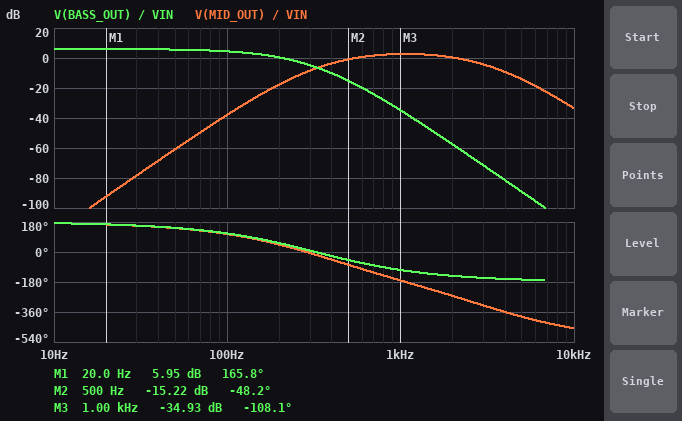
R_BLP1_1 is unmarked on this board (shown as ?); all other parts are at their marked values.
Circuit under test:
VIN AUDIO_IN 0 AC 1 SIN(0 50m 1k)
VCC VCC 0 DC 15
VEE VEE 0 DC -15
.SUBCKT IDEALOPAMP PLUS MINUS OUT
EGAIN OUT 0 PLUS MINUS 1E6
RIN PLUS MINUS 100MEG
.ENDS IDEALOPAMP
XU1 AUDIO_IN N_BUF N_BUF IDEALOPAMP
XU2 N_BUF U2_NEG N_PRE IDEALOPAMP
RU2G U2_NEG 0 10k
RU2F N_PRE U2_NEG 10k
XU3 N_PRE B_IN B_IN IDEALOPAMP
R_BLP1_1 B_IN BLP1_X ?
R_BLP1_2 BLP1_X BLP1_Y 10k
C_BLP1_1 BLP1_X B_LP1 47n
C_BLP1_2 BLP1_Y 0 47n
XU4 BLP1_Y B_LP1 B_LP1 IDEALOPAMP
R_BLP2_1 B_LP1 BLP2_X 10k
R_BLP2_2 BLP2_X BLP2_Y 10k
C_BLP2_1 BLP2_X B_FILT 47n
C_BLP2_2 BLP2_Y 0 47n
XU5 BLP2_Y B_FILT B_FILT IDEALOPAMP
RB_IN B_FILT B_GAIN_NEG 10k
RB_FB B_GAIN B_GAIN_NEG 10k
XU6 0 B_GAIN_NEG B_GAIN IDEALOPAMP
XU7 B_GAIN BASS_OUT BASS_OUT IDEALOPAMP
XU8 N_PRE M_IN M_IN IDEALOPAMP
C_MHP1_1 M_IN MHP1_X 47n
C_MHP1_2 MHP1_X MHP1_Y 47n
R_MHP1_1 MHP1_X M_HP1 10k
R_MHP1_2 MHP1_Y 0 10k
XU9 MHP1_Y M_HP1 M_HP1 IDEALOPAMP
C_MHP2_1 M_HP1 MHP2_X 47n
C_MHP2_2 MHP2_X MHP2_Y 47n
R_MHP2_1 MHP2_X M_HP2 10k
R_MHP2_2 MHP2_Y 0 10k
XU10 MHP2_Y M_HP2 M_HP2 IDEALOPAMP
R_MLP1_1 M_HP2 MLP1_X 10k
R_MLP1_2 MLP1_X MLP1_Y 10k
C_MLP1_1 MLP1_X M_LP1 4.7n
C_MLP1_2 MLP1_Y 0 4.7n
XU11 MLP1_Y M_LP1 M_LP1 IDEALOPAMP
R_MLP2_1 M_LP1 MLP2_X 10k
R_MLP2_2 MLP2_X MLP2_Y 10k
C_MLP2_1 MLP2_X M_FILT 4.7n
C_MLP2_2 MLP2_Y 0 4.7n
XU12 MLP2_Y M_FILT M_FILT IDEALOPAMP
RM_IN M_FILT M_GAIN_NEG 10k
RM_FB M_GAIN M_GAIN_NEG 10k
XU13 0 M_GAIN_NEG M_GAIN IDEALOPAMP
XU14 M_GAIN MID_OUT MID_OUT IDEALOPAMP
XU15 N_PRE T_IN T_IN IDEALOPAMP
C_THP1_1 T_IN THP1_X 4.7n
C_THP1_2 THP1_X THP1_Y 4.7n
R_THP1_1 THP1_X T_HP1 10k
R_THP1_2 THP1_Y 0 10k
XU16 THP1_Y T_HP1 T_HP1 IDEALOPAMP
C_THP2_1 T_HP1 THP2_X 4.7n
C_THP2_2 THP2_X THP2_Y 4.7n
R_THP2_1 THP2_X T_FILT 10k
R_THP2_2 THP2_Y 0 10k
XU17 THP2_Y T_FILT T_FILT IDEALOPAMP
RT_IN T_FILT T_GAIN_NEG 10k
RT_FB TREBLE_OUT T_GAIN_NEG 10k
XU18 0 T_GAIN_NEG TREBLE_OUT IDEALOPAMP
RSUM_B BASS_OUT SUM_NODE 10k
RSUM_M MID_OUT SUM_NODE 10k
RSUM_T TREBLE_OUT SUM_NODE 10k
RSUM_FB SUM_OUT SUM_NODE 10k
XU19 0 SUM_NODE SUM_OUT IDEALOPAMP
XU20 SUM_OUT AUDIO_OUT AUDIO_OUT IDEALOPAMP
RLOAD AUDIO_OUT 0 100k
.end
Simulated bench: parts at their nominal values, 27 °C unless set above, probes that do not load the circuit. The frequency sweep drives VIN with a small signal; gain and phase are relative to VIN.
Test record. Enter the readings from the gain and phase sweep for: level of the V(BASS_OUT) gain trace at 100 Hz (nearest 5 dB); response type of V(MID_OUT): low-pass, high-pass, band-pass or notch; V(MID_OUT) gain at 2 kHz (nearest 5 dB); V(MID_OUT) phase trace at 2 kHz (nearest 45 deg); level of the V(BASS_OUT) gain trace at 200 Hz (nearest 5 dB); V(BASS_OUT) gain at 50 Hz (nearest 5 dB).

5 dB
band-pass
0 dB
-270 deg
0 dB
5 dB
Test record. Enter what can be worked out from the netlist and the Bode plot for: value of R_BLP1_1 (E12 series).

12 kΩ
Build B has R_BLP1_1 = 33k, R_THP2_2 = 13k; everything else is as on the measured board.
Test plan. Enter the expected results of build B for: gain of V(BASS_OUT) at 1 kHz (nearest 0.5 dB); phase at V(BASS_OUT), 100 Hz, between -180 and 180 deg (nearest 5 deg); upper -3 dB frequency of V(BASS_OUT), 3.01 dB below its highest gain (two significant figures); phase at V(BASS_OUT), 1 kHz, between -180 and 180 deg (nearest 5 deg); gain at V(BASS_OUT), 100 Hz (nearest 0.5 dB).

-43.5 dB
85 deg
84 Hz
-120 deg
2.0 dB
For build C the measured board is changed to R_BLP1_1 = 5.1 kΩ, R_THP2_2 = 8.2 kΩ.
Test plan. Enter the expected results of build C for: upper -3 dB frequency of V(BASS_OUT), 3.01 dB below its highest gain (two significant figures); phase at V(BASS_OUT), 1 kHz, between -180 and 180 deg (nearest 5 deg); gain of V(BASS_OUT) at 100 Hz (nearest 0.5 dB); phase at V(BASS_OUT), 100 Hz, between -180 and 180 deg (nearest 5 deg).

160 Hz
-90 deg
5.0 dB
120 deg
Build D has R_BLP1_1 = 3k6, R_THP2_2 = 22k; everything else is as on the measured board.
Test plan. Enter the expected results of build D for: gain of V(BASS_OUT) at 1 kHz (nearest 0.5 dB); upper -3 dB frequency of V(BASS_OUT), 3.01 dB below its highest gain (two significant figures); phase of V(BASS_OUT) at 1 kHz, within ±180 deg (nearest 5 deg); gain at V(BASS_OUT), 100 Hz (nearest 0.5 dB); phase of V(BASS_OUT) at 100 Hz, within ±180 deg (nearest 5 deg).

-27.0 dB
170 Hz
-80 deg
5.0 dB
125 deg
